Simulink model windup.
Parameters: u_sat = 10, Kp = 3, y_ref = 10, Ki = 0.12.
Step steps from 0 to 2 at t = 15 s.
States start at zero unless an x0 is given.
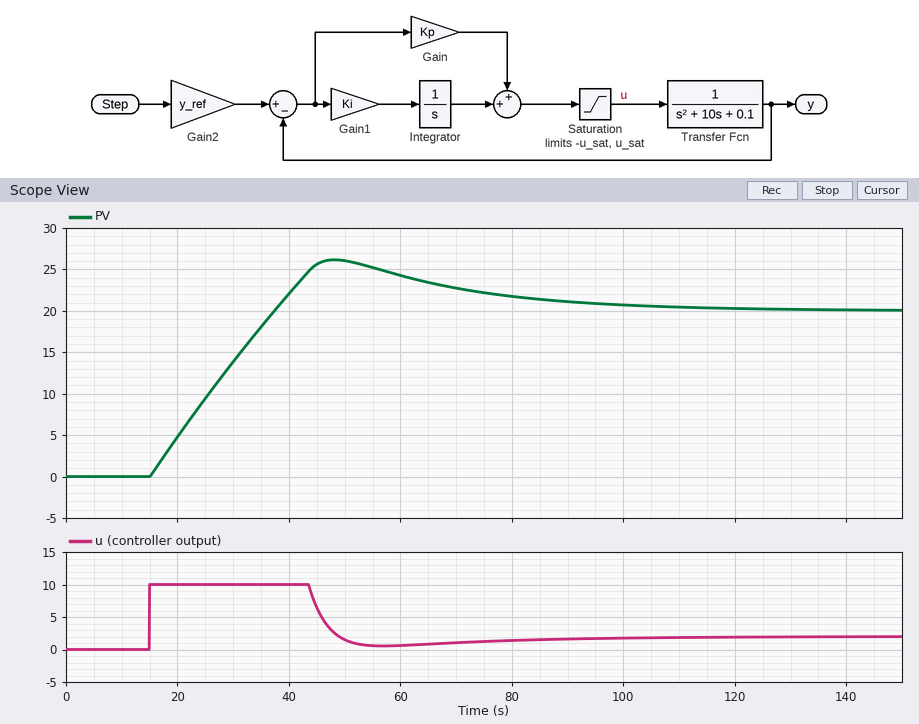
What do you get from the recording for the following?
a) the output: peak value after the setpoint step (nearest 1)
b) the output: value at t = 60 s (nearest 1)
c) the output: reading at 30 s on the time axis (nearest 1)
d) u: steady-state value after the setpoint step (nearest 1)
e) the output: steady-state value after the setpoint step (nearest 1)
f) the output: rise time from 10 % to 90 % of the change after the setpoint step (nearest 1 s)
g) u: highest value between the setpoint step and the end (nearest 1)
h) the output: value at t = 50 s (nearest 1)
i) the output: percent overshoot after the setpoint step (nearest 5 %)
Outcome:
26
24
14
2
20
18 s
10
26
30 %
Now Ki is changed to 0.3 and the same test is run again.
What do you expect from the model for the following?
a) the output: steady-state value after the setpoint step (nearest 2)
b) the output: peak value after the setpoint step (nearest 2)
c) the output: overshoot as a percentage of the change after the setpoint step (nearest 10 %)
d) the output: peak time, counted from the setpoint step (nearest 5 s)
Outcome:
20
32
60 %
40 s
